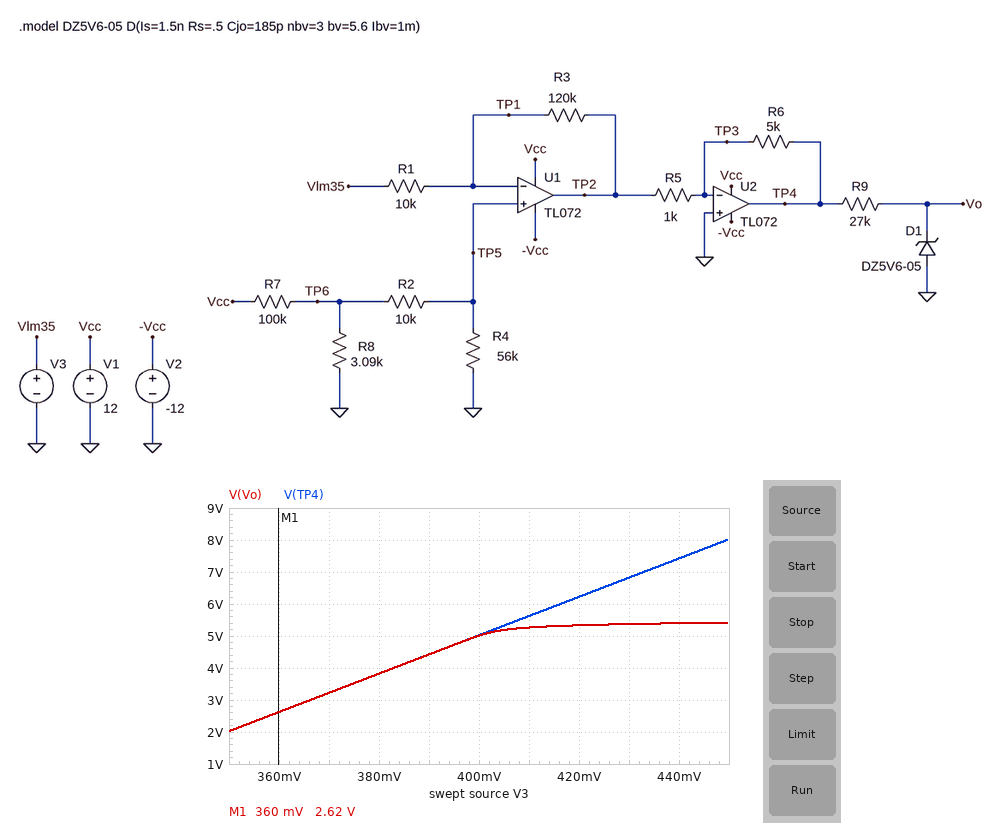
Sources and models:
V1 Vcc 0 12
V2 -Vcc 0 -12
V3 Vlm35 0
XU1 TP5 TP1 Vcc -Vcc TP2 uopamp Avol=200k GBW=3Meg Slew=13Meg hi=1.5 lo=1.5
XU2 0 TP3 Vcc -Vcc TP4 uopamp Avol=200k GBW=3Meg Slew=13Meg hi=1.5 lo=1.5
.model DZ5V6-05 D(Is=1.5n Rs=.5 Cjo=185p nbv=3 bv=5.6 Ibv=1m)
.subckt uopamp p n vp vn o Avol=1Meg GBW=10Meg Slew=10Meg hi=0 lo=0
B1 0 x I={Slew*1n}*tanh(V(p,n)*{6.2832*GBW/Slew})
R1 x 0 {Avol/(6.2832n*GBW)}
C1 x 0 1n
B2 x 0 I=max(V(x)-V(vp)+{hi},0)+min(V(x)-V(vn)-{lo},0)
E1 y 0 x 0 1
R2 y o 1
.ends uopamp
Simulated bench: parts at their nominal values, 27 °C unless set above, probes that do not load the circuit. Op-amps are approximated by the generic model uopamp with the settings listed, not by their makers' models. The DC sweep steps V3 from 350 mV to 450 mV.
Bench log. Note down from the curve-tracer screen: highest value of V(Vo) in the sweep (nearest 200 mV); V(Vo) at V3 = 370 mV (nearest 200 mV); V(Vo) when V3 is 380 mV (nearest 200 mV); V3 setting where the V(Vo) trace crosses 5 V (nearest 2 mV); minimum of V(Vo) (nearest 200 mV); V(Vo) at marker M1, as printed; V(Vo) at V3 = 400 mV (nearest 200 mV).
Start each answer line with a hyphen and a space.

- 5.4 V
- 3.2 V
- 3.8 V
- 400 mV
- 2.0 V
- 2.62 V
- 5.0 V
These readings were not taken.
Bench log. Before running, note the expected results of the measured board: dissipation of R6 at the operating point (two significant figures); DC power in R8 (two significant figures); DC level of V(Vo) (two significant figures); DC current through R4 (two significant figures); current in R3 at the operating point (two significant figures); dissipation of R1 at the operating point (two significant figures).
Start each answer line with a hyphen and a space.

- 28 mW
- 38 µW
- -320 mV
- 5.2 µA
- 29 µA
- 8.5 µW
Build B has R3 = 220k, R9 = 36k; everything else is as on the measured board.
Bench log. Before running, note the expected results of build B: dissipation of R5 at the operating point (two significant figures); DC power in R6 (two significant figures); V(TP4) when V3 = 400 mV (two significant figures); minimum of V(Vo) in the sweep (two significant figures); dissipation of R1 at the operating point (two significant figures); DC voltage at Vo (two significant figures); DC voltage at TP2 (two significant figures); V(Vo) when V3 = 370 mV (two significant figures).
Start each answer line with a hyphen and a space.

- 8.2 mW
- 41 mW
- 10 V
- 4.9 V
- 8.5 µW
- -310 mV
- 6.7 V
- 5.4 V
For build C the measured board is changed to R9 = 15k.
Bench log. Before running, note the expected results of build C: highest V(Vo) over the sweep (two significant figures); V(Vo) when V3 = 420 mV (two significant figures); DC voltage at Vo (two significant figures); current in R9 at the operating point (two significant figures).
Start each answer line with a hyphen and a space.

- 5.5 V
- 5.4 V
- -340 mV
- 680 µA
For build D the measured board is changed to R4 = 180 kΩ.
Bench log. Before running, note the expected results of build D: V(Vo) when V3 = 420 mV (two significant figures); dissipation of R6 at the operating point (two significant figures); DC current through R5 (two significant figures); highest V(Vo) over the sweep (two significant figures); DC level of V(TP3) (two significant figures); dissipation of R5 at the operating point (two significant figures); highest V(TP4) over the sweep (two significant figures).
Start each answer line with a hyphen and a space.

- 3.4 V
- 31 mW
- 2.5 mA
- 5.1 V
- 1.9 V
- 6.1 mW
- 5.2 V
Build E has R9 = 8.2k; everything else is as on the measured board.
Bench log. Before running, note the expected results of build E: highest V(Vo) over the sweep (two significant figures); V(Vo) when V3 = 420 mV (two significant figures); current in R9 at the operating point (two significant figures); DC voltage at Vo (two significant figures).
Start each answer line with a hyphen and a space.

- 5.5 V
- 5.4 V
- 1.2 mA
- -350 mV
